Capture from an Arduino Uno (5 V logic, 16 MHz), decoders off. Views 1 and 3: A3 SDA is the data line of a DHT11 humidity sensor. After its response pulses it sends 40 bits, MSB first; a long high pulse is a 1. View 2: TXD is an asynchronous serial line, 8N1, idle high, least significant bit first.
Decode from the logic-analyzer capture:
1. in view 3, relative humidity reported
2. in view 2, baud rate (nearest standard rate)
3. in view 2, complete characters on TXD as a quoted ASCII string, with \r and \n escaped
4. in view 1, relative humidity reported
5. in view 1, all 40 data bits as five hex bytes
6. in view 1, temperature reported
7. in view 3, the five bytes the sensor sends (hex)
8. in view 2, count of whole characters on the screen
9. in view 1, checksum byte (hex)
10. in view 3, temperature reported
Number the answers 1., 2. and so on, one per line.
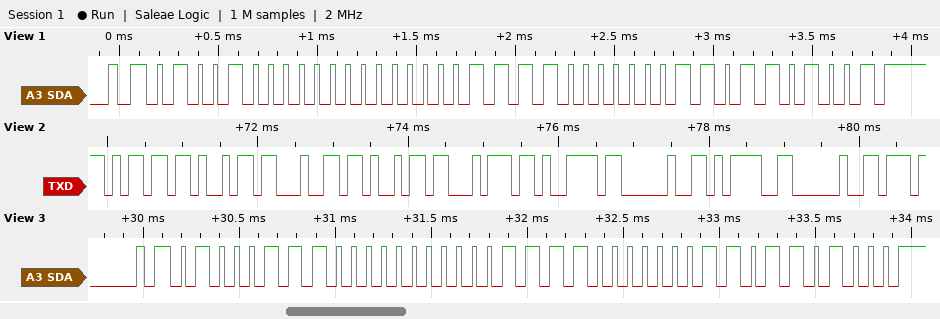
1. 71 %
2. 9600 baud
3. "midity = "
4. 72 %
5. 48 00 1E 03 69
6. 30.3 °C
7. 47 00 1E 03 68
8. 9
9. 0x69
10. 30.3 °C
